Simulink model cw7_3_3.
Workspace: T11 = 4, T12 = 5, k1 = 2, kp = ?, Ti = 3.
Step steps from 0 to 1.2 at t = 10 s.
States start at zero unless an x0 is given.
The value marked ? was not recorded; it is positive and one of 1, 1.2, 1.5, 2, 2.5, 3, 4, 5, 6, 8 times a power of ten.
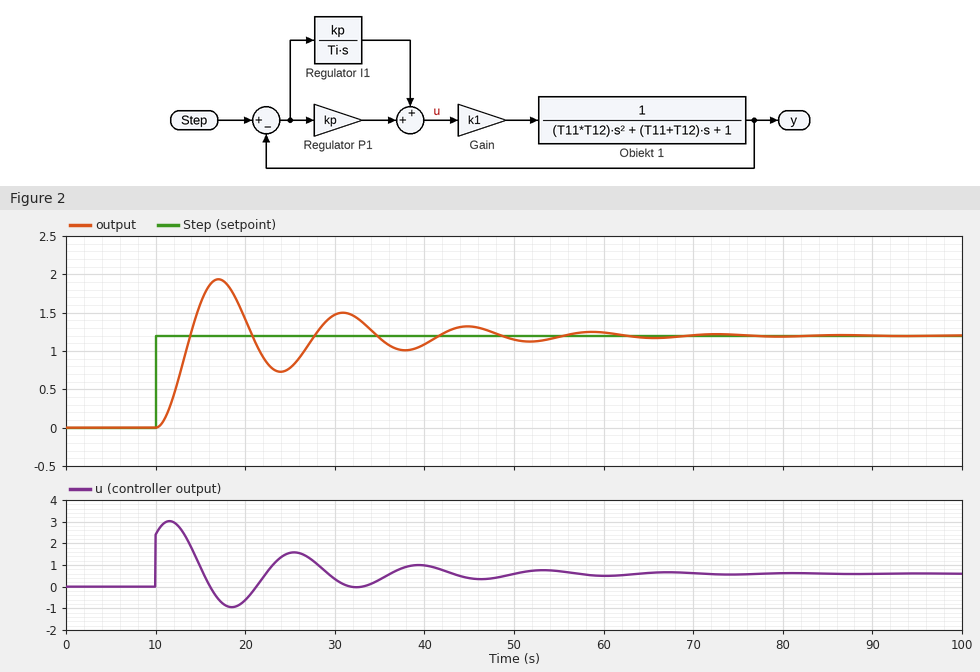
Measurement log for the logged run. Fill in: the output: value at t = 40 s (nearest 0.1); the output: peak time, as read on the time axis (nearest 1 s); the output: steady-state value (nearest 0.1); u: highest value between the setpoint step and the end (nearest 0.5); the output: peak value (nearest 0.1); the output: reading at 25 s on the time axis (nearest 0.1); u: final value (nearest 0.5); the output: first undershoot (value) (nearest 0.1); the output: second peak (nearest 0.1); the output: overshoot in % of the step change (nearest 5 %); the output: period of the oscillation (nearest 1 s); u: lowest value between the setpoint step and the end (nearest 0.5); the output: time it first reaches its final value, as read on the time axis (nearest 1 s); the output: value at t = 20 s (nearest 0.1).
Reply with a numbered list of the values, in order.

1. 1.1
2. 17 s
3. 1.2
4. 3.0
5. 1.9
6. 0.8
7. 0.5
8. 0.7
9. 1.5
10. 60 %
11. 14 s
12. -1.0
13. 14 s
14. 1.4
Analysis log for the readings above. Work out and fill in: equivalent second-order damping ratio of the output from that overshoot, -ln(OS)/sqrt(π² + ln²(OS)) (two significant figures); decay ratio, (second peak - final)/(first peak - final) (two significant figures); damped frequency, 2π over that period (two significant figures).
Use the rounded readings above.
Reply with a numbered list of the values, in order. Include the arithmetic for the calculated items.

1. ln(0.6) = -0.511; 0.511 / sqrt(9.870 + 0.261) = 0.16
2. (1.5 - 1.2) / (1.9 - 1.2) = 0.43
3. 2π / 14 = 0.45 rad/s
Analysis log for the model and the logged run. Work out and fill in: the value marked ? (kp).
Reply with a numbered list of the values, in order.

1. 2
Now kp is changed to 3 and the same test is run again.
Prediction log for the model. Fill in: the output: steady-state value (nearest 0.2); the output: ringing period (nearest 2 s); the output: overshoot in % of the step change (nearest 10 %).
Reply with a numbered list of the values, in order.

1. 1.2
2. 12 s
3. 70 %
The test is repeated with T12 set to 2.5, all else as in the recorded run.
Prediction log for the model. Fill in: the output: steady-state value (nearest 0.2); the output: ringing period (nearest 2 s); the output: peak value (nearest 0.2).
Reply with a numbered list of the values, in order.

1. 1.2
2. 10 s
3. 1.8
